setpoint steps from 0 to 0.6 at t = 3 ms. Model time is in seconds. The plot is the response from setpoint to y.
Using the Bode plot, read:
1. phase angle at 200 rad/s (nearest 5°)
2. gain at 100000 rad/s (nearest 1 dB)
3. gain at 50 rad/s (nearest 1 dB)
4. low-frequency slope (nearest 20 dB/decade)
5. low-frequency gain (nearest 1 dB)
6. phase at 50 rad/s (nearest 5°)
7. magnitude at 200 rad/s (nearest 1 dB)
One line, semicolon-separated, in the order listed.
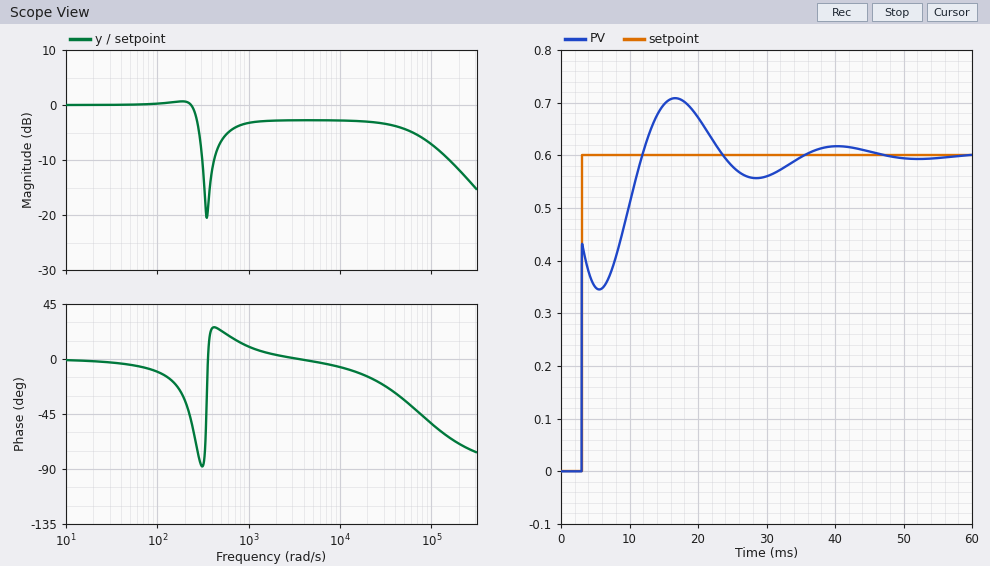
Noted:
-35°; -7 dB; 0 dB; 0 dB/decade; 0 dB; -5°; 1 dB
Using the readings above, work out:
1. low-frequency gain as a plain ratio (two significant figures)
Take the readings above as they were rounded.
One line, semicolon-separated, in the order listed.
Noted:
1.0
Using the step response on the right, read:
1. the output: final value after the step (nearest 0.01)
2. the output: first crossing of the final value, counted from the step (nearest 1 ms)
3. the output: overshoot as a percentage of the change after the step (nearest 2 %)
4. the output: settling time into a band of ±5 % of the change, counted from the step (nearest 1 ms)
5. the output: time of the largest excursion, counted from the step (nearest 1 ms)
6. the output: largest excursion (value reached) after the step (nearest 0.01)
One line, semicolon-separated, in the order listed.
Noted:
0.60; 9 ms; 18 %; 29 ms; 14 ms; 0.71
